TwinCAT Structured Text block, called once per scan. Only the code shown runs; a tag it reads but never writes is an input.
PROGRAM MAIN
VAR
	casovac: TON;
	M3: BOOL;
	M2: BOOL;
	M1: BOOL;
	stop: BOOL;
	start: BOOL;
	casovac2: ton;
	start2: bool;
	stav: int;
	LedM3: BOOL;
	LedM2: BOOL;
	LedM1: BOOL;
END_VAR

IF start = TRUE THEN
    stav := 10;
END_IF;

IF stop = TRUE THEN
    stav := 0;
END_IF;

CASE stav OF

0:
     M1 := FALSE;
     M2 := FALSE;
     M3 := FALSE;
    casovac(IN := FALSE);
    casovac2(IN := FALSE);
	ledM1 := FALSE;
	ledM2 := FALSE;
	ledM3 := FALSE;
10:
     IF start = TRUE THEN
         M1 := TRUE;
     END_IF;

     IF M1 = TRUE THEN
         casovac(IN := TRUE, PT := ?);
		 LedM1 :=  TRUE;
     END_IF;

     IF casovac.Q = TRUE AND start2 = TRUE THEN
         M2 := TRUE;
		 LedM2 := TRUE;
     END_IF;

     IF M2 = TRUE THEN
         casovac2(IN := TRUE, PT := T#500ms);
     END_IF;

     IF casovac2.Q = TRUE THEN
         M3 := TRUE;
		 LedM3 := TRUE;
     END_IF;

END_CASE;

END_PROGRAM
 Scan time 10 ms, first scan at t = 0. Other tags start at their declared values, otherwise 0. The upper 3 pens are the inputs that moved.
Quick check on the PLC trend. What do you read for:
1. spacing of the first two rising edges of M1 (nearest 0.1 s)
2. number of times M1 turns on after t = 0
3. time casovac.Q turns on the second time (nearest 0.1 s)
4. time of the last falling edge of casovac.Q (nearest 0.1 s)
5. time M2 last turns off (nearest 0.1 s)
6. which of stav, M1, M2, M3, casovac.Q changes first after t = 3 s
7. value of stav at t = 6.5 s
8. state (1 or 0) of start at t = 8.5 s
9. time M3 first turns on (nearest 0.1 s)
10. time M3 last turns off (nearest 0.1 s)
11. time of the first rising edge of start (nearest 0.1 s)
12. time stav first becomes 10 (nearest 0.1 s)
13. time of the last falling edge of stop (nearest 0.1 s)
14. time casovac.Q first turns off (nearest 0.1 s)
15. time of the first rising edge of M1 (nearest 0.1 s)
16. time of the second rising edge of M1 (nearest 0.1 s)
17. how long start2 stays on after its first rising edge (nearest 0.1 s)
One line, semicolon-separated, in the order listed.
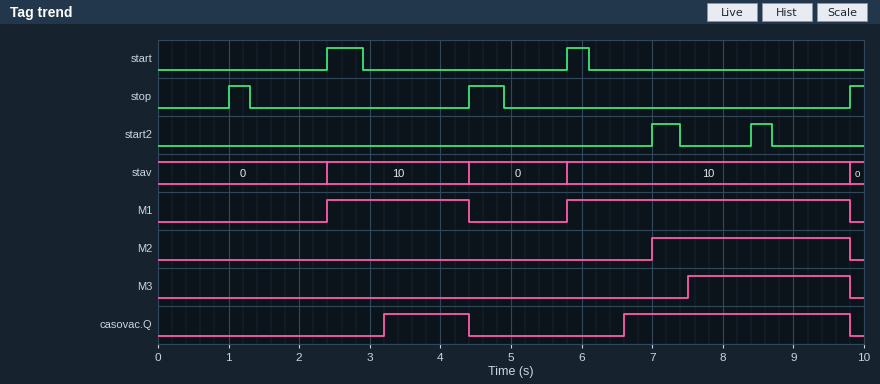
3.4 s; 2; 6.6 s; 9.8 s; 9.8 s; casovac.Q; 10; 0; 7.5 s; 9.8 s; 2.4 s; 2.4 s; 4.9 s; 4.4 s; 2.4 s; 5.8 s; 0.4 s
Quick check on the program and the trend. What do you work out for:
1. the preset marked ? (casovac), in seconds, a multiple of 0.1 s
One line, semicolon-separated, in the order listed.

0.8 s
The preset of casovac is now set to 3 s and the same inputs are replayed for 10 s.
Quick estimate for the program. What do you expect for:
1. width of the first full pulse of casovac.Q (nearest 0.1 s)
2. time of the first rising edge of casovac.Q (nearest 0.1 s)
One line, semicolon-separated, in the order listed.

1.0 s; 8.8 s
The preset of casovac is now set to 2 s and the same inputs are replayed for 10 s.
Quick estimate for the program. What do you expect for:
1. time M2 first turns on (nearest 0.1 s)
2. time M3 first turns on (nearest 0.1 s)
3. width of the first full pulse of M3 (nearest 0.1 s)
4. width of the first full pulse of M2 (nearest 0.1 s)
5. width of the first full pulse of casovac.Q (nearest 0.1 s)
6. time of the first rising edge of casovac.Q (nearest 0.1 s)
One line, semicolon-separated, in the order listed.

8.4 s; 8.9 s; 0.9 s; 1.4 s; 2.0 s; 7.8 s
